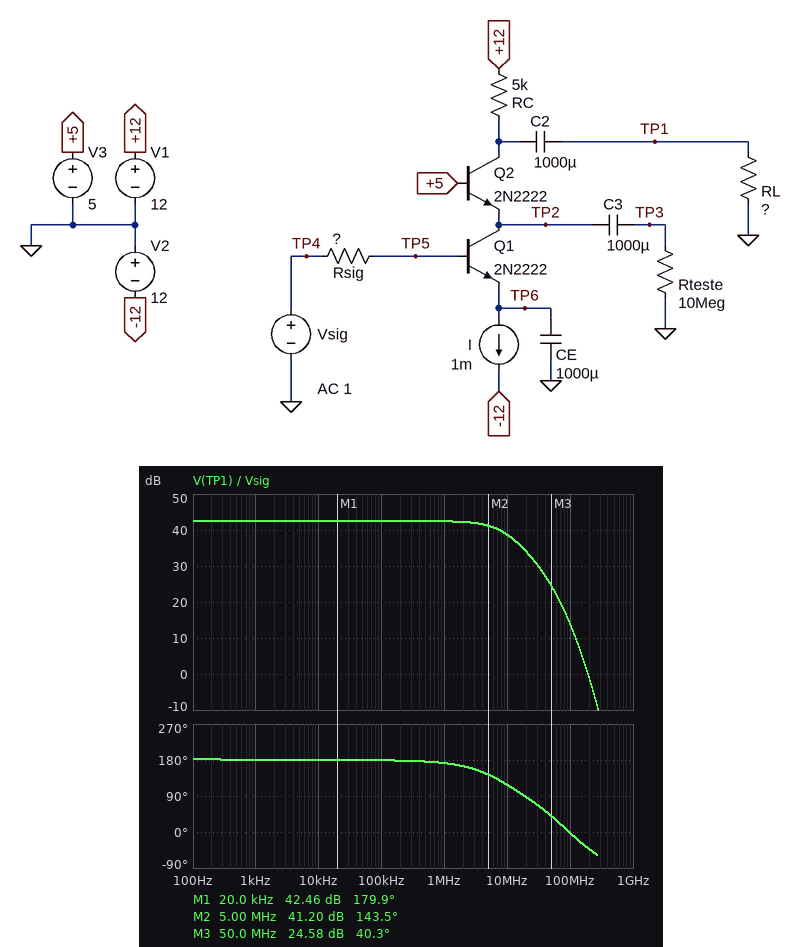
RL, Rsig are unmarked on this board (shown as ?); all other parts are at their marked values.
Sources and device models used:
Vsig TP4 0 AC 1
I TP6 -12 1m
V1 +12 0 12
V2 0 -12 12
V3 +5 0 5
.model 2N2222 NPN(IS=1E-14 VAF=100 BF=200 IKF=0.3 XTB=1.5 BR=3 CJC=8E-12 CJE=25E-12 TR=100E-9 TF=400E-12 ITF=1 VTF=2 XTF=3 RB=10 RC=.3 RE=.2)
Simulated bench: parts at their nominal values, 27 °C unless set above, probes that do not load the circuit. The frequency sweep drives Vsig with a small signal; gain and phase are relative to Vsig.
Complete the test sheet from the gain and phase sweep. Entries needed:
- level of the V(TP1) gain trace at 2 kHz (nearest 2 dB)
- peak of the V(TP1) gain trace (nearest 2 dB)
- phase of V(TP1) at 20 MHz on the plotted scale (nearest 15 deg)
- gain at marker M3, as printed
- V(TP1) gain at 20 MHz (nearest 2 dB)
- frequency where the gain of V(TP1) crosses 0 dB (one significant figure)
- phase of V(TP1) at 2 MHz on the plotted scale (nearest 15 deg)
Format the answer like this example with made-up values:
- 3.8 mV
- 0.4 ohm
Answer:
- 42 dB
- 42 dB
- 90 deg
- 24.58 dB
- 34 dB
- 200 MHz
- 165 deg
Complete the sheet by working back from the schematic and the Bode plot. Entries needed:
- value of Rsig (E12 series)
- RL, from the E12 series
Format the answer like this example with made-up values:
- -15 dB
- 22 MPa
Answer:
- 22 Ω
- 12 kΩ
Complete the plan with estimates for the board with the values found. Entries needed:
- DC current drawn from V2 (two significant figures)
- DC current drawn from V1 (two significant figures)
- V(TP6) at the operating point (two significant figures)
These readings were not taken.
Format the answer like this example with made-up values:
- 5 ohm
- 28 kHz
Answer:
- 1.0 mA
- 990 µA
- -650 mV
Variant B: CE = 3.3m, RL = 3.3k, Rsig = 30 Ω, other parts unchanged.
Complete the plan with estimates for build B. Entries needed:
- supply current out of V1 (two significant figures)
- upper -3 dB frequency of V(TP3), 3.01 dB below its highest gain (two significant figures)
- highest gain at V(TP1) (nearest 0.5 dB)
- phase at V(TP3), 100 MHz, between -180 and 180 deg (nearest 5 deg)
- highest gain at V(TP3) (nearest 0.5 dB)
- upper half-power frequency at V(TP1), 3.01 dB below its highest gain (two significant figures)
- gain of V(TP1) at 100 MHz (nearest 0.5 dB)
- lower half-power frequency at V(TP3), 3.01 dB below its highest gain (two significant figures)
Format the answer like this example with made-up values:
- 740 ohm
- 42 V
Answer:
- 990 µA
- 62 MHz
- 37.5 dB
- 90 deg
- 1.5 dB
- 14 MHz
- 12.5 dB
- 2.7 Hz
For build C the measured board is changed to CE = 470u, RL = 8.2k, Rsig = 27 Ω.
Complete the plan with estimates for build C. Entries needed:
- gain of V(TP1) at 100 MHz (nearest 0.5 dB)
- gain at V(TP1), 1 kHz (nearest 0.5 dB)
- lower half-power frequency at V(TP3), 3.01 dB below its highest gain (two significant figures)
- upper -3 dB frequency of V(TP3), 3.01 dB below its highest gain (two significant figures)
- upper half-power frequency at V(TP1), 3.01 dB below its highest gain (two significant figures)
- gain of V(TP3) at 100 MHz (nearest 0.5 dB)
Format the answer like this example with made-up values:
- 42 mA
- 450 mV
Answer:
- 13.0 dB
- 41.5 dB
- 22 Hz
- 61 MHz
- 9.6 MHz
- -5.0 dB
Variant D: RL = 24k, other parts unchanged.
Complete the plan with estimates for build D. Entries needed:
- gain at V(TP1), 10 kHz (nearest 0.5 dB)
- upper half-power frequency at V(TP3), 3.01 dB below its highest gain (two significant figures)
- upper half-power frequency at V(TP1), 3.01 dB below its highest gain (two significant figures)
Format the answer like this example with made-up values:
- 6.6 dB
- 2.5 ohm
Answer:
- 44.0 dB
- 64 MHz
- 7.3 MHz
